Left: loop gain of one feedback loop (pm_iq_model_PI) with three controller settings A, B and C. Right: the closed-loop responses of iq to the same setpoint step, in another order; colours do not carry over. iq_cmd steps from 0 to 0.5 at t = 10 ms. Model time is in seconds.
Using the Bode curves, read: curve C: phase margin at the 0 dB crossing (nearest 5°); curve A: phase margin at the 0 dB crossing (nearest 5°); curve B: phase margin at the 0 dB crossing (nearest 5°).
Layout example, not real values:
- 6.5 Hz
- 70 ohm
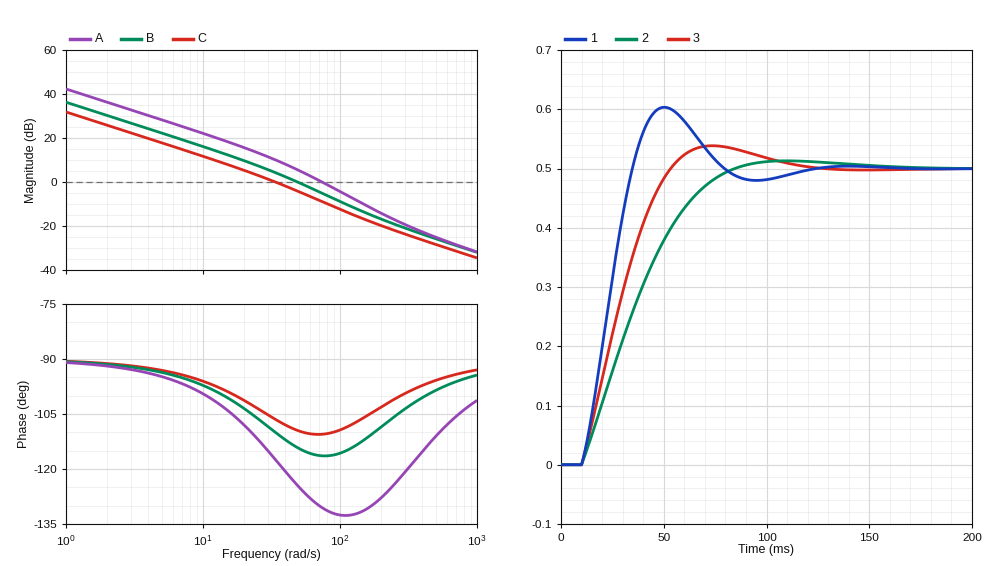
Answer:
- 75°
- 50°
- 65°
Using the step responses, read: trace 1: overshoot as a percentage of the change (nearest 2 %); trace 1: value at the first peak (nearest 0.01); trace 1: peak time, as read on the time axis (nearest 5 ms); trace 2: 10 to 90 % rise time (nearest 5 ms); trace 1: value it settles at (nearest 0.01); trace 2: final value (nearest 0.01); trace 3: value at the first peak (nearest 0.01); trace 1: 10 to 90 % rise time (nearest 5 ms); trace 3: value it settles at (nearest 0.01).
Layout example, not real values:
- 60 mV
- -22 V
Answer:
- 20 %
- 0.60
- 50 ms
- 50 ms
- 0.50
- 0.50
- 0.54
- 20 ms
- 0.50
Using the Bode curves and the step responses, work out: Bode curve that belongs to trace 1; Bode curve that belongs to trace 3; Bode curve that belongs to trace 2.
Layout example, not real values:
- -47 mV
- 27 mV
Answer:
- A
- B
- C
